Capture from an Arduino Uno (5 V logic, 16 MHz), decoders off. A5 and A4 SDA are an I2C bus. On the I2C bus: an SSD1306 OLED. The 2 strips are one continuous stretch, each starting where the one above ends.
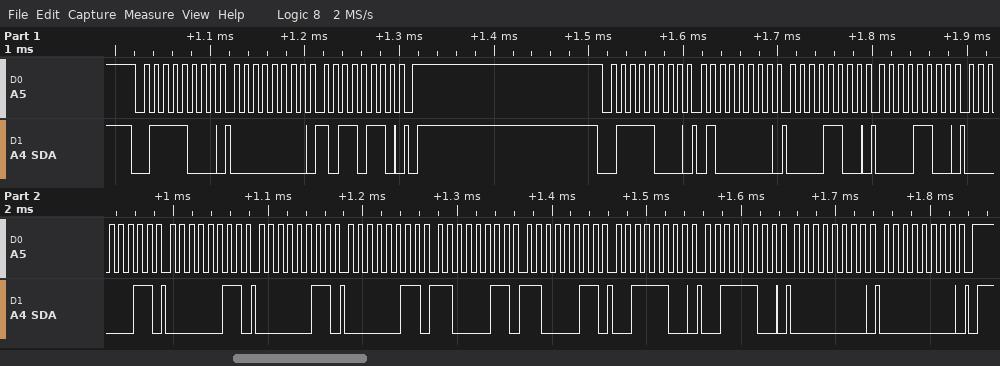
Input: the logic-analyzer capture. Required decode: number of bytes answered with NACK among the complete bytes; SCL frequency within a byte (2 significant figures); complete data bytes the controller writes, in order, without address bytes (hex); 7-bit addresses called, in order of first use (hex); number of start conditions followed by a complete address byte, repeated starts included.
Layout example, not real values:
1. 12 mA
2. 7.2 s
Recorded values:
1. 0
2. 100 kHz
3. 00 B6 40 0C 0C 03 03 03 03 C3 C3 3C 3C 00 00
4. 0x3C
5. 2
